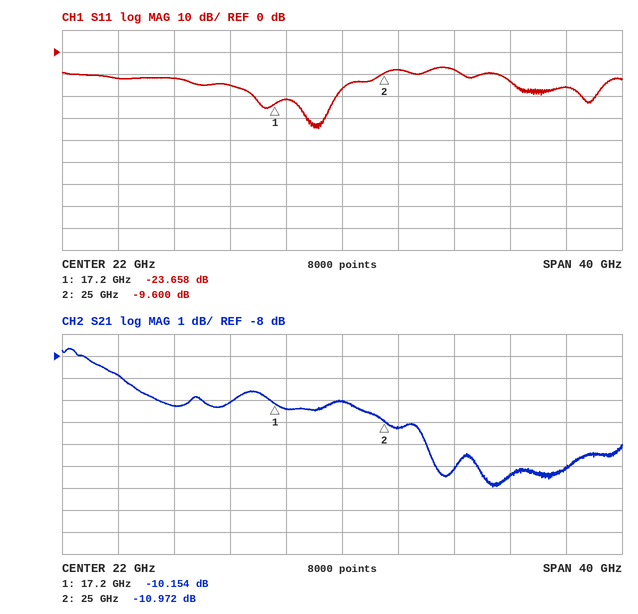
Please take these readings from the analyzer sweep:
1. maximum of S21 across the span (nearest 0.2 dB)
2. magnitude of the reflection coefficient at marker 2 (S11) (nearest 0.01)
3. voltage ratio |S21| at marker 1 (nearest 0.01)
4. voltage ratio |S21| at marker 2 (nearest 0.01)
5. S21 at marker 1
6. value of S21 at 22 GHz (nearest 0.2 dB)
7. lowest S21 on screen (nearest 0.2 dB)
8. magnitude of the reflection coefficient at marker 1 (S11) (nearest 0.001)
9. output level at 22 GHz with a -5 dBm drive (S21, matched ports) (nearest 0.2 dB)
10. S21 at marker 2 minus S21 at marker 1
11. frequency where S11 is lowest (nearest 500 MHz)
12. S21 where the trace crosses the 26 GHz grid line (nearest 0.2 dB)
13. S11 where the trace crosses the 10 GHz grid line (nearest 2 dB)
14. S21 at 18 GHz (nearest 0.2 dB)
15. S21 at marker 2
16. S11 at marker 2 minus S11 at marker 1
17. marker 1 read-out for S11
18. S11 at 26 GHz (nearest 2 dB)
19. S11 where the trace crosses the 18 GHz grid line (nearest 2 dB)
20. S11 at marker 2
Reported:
-7.6 dB
0.33
0.31
0.28
-10.154 dB
-10.0 dB
-14.0 dB
0.066
-15.0 dBm
-0.818 dB
20.5 GHz
-11.2 dB
-12 dB
-10.4 dB
-10.972 dB
14.058 dB
-23.658 dB
-8 dB
-22 dB
-9.600 dB
